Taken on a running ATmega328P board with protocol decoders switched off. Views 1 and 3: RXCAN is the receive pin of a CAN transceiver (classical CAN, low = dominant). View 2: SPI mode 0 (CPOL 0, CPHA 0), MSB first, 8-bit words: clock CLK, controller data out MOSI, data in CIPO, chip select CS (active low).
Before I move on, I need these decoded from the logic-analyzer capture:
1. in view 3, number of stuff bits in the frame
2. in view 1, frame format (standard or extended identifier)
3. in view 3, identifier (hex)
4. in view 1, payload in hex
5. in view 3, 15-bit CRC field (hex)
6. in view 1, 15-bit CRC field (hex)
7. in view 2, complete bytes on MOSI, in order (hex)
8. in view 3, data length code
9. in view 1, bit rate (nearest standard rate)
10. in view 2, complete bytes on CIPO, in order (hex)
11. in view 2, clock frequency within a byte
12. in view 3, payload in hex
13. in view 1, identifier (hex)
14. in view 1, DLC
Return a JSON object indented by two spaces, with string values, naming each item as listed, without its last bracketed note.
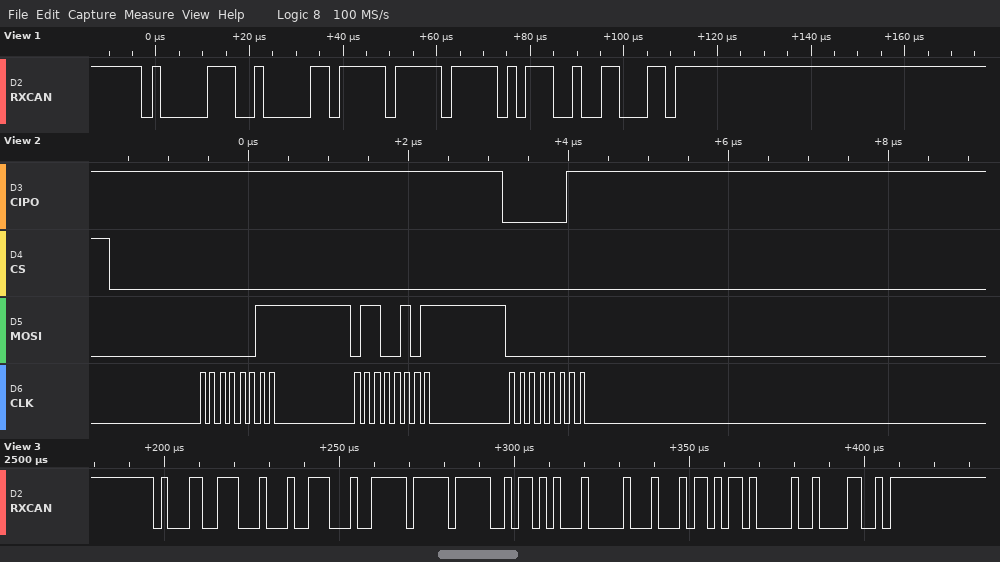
{
  "in view 3, number of stuff bits in the frame": "5",
  "in view 1, frame format": "standard",
  "in view 3, identifier": "0x467",
  "in view 1, payload in hex": "FF FF",
  "in view 3, 15-bit CRC field": "0x010C",
  "in view 1, 15-bit CRC field": "0x3931",
  "in view 2, complete bytes on MOSI, in order": "0x03 0x65 0x00",
  "in view 3, data length code": "8",
  "in view 1, bit rate": "500 kbit/s",
  "in view 2, complete bytes on CIPO, in order": "0xFF 0xFF 0x03",
  "in view 2, clock frequency within a byte": "8 MHz",
  "in view 3, payload in hex": "9C 4F FF EB 51 00 8B 5A",
  "in view 1, identifier": "0x419",
  "in view 1, DLC": "2"
}
